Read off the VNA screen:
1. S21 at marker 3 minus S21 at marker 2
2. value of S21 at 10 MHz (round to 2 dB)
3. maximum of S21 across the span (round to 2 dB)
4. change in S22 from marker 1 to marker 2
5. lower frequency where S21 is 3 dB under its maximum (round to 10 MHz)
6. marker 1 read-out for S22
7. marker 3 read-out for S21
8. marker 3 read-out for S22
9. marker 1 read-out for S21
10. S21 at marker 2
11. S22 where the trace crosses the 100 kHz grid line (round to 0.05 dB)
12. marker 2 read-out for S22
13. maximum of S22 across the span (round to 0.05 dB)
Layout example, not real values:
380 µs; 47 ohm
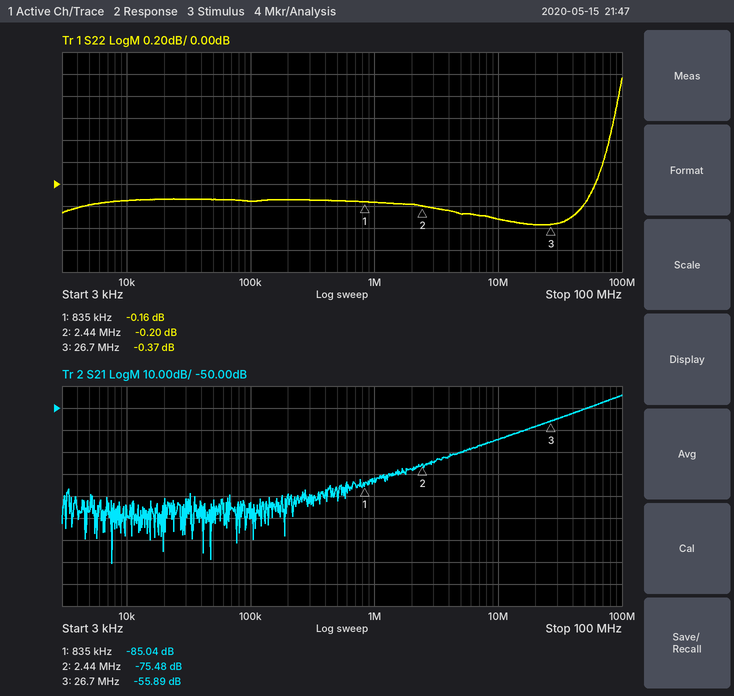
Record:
19.59 dB; -64 dB; -44 dB; -0.04 dB; 70 MHz; -0.16 dB; -55.89 dB; -0.37 dB; -85.04 dB; -75.48 dB; -0.15 dB; -0.20 dB; 0.95 dB
